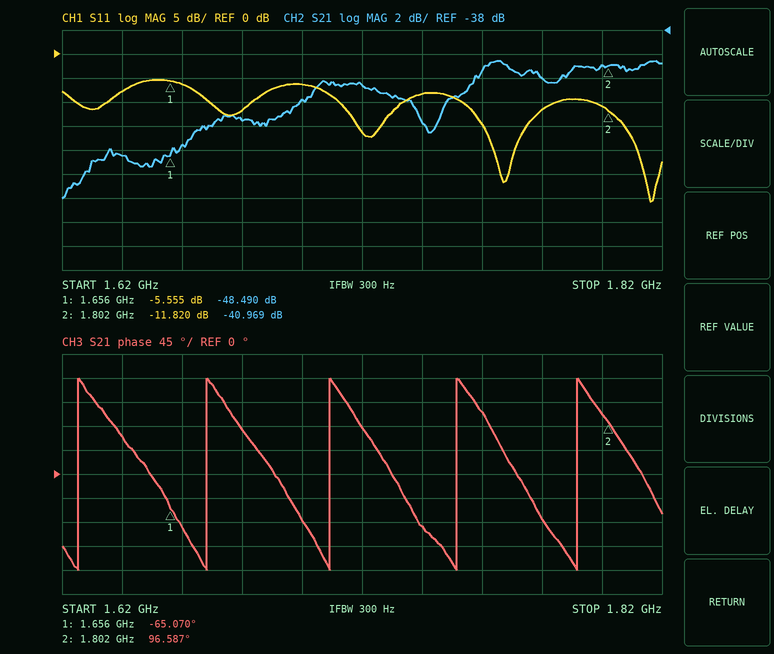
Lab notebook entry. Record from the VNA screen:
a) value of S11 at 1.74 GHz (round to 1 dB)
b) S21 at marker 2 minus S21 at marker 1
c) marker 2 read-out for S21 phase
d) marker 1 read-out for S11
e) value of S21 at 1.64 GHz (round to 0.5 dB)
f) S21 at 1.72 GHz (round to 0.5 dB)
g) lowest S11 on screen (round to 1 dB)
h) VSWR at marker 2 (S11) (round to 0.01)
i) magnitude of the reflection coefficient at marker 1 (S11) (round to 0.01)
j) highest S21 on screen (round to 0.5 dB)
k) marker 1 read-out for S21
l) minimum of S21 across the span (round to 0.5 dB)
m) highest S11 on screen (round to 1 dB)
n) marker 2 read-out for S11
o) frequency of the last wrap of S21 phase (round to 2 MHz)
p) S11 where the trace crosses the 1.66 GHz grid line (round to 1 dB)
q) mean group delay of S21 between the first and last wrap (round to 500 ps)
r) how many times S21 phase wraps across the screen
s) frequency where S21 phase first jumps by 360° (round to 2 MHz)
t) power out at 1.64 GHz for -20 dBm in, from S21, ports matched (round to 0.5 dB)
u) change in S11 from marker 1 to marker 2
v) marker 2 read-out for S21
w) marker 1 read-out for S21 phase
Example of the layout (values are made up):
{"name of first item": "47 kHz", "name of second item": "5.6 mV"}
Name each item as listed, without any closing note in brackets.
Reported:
{"value of S11 at 1.74 GHz": "-8 dB", "S21 at marker 2 minus S21 at marker 1": "7.521 dB", "marker 2 read-out for S21 phase": "96.587°", "marker 1 read-out for S11": "-5.555 dB", "value of S21 at 1.64 GHz": "-48.5 dB", "S21 at 1.72 GHz": "-42.5 dB", "lowest S11 on screen": "-31 dB", "VSWR at marker 2 (S11)": "1.69", "magnitude of the reflection coefficient at marker 1 (S11)": "0.53", "highest S21 on screen": "-40.5 dB", "marker 1 read-out for S21": "-48.490 dB", "minimum of S21 across the span": "-52.0 dB", "highest S11 on screen": "-5 dB", "marker 2 read-out for S11": "-11.820 dB", "frequency of the last wrap of S21 phase": "1.792 GHz", "S11 where the trace crosses the 1.66 GHz grid line": "-6 dB", "mean group delay of S21 between the first and last wrap": "24.0 ns", "how many times S21 phase wraps across the screen": "5", "frequency where S21 phase first jumps by 360°": "1.626 GHz", "power out at 1.64 GHz for -20 dBm in, from S21, ports matched": "-68.5 dBm", "change in S11 from marker 1 to marker 2": "-6.265 dB", "marker 2 read-out for S21": "-40.969 dB", "marker 1 read-out for S21 phase": "-65.070°"}
